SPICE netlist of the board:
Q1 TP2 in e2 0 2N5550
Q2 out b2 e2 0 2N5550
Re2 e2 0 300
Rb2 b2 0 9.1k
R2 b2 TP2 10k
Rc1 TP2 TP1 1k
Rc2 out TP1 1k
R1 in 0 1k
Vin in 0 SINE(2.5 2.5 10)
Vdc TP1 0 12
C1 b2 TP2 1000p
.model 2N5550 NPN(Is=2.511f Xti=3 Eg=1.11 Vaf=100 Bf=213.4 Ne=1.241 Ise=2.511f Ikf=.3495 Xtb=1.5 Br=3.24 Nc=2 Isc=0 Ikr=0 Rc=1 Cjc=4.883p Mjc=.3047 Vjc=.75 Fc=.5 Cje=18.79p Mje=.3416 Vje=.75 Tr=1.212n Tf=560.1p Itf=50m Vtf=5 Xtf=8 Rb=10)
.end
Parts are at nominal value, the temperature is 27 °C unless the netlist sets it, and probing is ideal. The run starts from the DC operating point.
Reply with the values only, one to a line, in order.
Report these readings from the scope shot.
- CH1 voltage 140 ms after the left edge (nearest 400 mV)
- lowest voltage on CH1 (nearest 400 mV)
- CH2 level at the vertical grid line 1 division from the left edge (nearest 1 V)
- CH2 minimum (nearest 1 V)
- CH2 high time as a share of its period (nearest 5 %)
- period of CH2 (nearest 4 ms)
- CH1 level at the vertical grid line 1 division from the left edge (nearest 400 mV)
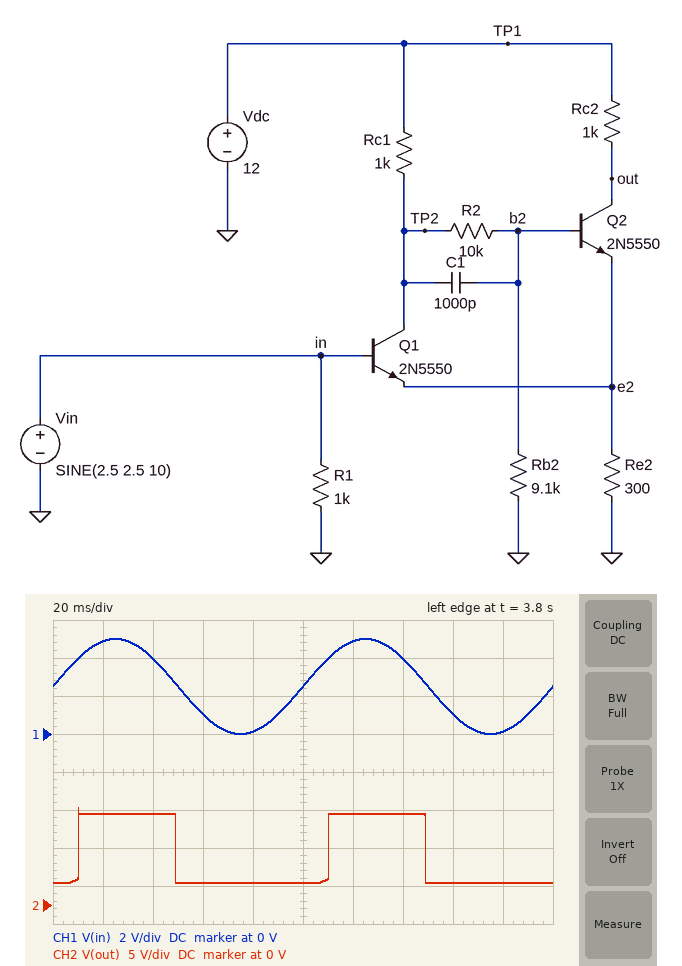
4.0 V
0 V
12 V
3 V
40 %
100 ms
4.8 V
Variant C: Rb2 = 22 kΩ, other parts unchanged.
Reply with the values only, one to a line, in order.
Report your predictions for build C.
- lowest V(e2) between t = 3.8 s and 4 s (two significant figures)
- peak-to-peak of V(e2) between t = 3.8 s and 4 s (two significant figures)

2.3 V
1.8 V
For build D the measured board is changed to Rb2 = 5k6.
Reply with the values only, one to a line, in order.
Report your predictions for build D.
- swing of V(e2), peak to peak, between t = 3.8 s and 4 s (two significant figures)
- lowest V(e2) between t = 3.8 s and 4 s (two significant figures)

2.5 V
1.6 V
